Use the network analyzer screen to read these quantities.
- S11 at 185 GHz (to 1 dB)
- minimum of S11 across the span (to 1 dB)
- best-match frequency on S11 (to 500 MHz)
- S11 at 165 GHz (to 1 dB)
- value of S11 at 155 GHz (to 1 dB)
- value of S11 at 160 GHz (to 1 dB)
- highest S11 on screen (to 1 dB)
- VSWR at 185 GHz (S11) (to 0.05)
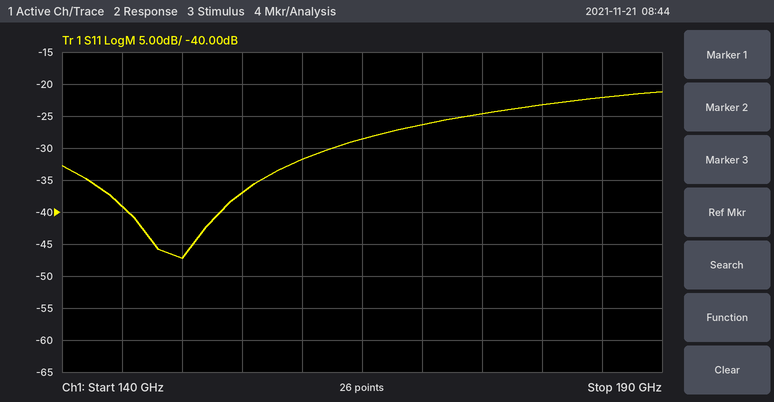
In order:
-22 dB
-47 dB
150.0 GHz
-29 dB
-37 dB
-32 dB
-21 dB
1.15
